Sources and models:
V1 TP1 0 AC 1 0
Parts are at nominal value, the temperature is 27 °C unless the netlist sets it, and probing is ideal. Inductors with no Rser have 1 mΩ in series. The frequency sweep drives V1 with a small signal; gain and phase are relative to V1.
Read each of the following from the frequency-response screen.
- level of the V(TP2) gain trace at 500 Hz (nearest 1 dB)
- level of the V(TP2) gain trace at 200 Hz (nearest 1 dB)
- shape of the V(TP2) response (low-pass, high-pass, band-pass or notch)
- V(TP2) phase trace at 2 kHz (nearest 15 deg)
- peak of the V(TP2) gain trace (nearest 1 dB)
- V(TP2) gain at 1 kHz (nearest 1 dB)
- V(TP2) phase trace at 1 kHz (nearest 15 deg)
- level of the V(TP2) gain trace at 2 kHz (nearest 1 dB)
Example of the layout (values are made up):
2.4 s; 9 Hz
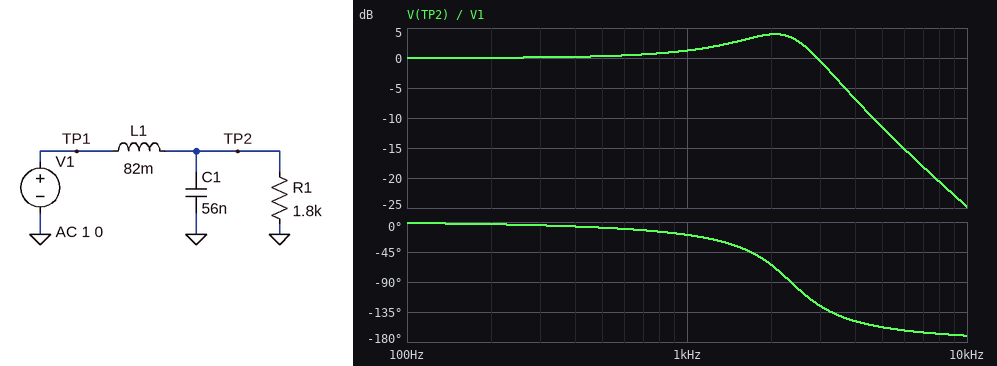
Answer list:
0 dB; 0 dB; low-pass; -60 deg; 4 dB; 1 dB; -15 deg; 4 dB
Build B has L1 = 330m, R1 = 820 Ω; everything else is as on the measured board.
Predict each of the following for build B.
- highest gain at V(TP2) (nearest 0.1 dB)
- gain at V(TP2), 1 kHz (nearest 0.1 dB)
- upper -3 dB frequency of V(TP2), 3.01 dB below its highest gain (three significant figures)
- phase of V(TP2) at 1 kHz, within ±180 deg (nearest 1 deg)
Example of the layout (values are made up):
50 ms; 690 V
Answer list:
0 dB; -8.1 dB; 445 Hz; -84 deg
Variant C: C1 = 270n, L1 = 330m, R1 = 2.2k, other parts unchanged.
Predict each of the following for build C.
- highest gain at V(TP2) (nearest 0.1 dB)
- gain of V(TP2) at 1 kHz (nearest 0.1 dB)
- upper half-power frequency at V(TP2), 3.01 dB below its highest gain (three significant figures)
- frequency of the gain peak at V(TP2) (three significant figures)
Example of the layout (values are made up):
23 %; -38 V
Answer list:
6.3 dB; -8.6 dB; 622 Hz; 498 Hz
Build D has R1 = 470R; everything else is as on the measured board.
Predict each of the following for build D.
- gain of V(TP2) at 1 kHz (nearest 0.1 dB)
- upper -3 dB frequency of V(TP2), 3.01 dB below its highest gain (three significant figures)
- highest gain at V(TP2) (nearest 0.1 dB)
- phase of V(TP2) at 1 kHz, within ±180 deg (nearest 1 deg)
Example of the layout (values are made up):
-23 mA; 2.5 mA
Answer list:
-2.7 dB; 1.07 kHz; 0 dB; -53 deg
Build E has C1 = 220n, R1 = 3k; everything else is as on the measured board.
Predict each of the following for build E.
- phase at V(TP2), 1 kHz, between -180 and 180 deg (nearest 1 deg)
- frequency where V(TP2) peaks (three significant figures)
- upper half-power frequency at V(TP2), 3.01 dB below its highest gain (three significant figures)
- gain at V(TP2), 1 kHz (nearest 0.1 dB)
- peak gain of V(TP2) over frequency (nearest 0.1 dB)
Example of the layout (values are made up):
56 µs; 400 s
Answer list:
-31 deg; 1.17 kHz; 1.29 kHz; 9.5 dB; 13.9 dB
